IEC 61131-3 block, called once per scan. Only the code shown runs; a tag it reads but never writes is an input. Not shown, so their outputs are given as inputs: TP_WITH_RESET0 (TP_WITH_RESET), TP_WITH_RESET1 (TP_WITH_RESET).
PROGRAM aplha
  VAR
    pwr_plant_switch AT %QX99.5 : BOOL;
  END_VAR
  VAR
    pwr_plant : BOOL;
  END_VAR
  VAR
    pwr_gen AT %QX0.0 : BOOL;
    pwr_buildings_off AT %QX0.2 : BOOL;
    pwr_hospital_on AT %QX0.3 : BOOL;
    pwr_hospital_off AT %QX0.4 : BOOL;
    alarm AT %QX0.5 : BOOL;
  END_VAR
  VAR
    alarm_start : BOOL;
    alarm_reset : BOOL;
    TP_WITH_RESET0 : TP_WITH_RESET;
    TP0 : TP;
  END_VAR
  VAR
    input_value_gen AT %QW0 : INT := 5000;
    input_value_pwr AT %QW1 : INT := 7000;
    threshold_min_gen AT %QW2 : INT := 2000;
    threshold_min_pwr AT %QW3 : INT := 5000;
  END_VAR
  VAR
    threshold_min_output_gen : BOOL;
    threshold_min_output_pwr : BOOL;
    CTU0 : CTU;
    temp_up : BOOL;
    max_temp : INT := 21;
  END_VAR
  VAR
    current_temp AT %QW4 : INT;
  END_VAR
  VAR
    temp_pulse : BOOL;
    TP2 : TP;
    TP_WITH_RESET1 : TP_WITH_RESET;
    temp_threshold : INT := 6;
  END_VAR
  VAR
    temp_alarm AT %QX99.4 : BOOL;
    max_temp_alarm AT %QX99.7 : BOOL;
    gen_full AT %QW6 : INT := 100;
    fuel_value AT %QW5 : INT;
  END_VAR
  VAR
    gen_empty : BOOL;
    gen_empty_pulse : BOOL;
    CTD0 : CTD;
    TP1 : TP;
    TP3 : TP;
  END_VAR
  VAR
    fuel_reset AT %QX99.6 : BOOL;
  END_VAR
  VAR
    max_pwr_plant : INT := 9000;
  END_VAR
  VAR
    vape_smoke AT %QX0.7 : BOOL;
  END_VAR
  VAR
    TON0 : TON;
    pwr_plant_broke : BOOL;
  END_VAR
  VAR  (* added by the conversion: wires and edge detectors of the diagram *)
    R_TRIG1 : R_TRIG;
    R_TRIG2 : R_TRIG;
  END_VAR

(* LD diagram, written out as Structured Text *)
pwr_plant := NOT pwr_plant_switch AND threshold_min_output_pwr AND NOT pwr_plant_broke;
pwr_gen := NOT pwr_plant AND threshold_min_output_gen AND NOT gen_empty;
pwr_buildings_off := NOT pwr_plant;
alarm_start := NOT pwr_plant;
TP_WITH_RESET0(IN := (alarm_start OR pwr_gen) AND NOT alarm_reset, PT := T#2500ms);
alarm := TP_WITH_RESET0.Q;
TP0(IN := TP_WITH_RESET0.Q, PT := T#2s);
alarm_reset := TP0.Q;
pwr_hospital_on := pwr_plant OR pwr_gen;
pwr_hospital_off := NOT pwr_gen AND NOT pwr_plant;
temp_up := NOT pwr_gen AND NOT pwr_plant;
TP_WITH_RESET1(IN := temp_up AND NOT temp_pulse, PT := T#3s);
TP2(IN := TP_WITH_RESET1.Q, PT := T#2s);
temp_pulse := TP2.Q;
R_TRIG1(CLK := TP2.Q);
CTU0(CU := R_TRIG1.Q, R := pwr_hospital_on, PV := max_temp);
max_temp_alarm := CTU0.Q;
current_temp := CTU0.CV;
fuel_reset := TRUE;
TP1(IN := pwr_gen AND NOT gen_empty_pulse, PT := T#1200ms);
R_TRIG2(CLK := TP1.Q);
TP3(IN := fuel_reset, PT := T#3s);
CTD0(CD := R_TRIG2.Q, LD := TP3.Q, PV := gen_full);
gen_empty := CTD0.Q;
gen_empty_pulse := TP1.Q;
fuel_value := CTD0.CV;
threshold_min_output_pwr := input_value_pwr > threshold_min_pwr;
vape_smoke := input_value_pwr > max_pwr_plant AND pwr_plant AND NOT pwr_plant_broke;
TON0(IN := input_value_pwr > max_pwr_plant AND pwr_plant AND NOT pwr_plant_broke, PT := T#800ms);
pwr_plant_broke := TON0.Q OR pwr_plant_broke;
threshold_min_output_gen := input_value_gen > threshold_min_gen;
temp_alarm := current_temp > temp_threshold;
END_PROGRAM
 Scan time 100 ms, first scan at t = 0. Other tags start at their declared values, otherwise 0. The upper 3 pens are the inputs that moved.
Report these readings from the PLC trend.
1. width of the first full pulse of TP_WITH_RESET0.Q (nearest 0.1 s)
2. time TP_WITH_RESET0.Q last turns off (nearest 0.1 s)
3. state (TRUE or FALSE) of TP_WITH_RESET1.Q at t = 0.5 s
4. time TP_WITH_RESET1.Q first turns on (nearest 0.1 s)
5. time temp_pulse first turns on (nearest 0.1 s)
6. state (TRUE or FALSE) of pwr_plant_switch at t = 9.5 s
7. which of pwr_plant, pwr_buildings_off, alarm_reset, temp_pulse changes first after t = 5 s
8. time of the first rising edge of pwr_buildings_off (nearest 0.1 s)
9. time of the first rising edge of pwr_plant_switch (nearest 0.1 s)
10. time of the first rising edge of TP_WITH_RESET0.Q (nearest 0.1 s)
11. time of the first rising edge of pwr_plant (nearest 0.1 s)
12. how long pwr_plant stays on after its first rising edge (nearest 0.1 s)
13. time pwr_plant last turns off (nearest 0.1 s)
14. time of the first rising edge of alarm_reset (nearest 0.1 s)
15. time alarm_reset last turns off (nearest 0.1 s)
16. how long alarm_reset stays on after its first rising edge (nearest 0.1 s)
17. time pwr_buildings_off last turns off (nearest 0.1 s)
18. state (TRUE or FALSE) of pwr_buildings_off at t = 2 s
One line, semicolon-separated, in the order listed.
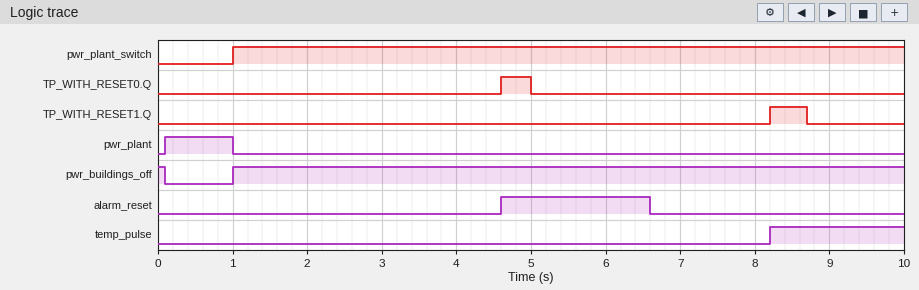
0.4 s; 5.0 s; FALSE; 8.2 s; 8.2 s; TRUE; alarm_reset; 1.0 s; 1.0 s; 4.6 s; 0.1 s; 0.9 s; 1.0 s; 4.6 s; 6.6 s; 2.0 s; 0.1 s; TRUE
